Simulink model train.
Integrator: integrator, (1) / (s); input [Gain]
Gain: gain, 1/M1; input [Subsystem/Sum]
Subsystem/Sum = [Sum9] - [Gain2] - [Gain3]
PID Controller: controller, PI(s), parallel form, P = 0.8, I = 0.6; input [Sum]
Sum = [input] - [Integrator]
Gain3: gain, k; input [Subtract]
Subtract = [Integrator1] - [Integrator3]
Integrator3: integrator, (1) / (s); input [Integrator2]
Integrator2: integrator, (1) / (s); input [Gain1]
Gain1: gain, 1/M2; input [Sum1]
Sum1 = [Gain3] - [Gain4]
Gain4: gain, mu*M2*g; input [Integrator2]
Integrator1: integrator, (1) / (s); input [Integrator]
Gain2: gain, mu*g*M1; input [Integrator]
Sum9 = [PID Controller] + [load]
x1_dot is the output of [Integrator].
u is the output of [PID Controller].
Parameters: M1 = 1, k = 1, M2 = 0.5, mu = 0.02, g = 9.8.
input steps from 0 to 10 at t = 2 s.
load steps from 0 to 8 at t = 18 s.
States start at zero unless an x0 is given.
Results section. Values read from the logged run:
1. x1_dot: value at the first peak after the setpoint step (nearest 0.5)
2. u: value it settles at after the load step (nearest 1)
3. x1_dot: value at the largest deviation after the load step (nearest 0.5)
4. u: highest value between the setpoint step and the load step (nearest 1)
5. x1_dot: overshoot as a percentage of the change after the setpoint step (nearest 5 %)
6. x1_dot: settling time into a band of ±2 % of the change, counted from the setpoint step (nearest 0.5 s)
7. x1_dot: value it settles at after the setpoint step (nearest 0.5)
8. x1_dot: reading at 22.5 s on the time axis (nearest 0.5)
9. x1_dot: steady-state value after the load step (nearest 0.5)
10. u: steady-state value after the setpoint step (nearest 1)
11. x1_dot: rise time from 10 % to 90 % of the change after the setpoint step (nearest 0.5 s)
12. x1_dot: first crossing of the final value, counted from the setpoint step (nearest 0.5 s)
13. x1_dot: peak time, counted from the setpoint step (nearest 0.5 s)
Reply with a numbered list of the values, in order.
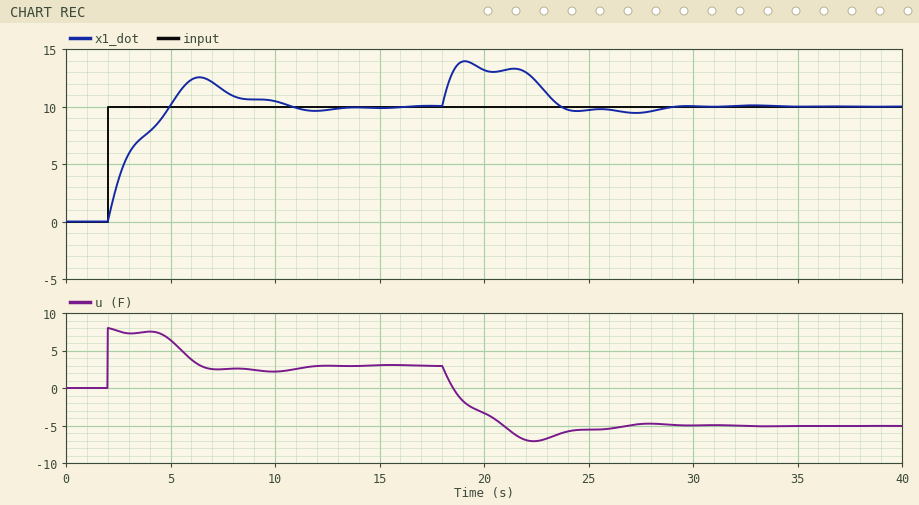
1. 12.5
2. -5
3. 14.0
4. 8
5. 25 %
6. 11.0 s
7. 10.0
8. 12.0
9. 10.0
10. 3
11. 2.5 s
12. 3.0 s
13. 4.5 s
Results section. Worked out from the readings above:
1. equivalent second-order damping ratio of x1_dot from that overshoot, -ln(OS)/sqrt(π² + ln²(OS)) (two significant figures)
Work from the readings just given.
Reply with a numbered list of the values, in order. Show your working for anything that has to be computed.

1. ln(0.25) = -1.386; 1.386 / sqrt(9.870 + 1.922) = 0.40
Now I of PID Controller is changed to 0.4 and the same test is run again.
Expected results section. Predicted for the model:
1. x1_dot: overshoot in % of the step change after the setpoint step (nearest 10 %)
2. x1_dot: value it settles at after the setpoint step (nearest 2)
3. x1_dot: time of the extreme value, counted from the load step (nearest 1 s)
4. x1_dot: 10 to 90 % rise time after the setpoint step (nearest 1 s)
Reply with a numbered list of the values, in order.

1. 20 %
2. 10
3. 4 s
4. 3 s
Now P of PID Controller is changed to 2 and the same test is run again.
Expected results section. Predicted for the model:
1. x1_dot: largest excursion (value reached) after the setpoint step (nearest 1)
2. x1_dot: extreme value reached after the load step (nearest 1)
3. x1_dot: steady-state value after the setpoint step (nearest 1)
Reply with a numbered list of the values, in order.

1. 11
2. 13
3. 10
